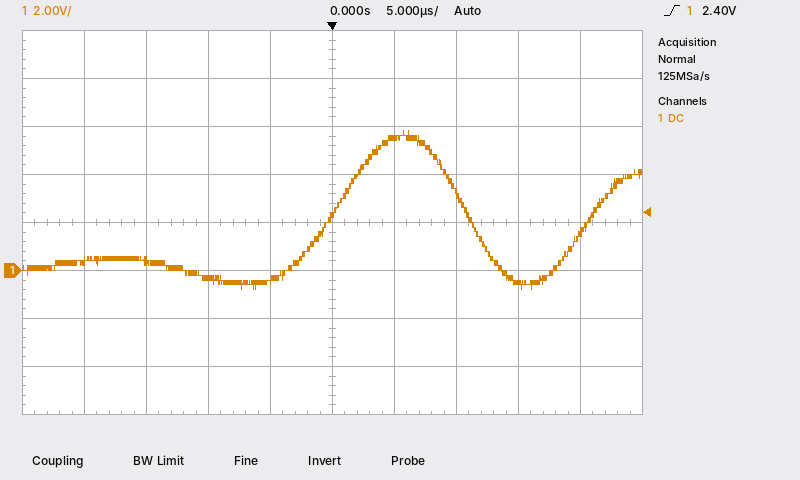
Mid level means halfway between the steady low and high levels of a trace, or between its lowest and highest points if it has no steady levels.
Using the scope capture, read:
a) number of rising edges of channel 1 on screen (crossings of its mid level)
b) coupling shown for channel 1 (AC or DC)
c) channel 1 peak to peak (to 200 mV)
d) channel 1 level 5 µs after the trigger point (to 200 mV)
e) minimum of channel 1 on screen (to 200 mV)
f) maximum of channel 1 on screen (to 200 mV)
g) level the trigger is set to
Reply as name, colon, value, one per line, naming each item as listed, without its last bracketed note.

number of rising edges of channel 1 on screen: 2
coupling shown for channel 1: DC
channel 1 peak to peak: 6.6 V
channel 1 level 5 µs after the trigger point: 5.6 V
minimum of channel 1 on screen: -800 mV
maximum of channel 1 on screen: 5.8 V
level the trigger is set to: 2.40 V
